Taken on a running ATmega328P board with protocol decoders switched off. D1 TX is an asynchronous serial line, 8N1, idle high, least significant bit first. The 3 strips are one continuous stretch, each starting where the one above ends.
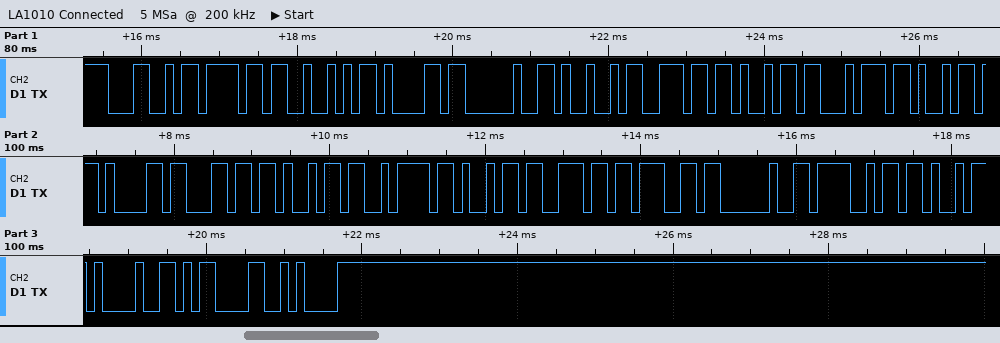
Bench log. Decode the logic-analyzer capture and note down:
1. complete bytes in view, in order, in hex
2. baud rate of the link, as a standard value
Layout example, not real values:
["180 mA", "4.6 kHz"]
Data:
["4C 6F 52 61 20 49 6E 69 74 69 61 6C 69 7A 69 6E 67 20 4F 4B 21 0D 0A", "9600 baud"]
